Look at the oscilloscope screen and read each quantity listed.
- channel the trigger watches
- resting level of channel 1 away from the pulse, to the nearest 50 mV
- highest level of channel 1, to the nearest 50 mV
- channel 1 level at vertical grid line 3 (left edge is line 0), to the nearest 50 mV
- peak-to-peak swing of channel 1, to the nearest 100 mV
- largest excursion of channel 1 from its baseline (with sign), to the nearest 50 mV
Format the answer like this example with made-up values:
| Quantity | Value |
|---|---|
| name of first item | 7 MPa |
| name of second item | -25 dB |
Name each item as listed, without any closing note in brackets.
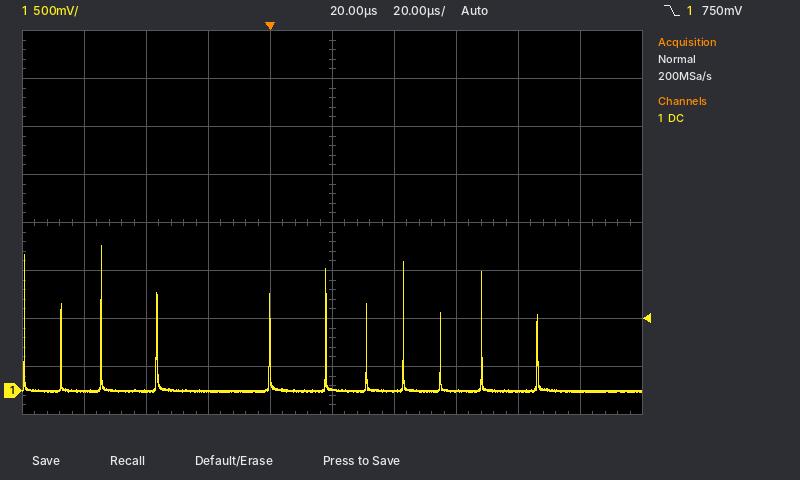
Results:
| Quantity | Value |
|---|---|
| channel the trigger watches | channel 1 |
| resting level of channel 1 away from the pulse, to the nearest 50 mV | 0 mV |
| highest level of channel 1, to the nearest 50 mV | 1.50 V |
| channel 1 level at vertical grid line 3 (left edge is line 0), to the nearest 50 mV | 0 mV |
| peak-to-peak swing of channel 1, to the nearest 100 mV | 1.50 V |
| largest excursion of channel 1 from its baseline (with sign), to the nearest 50 mV | +1.50 V |
